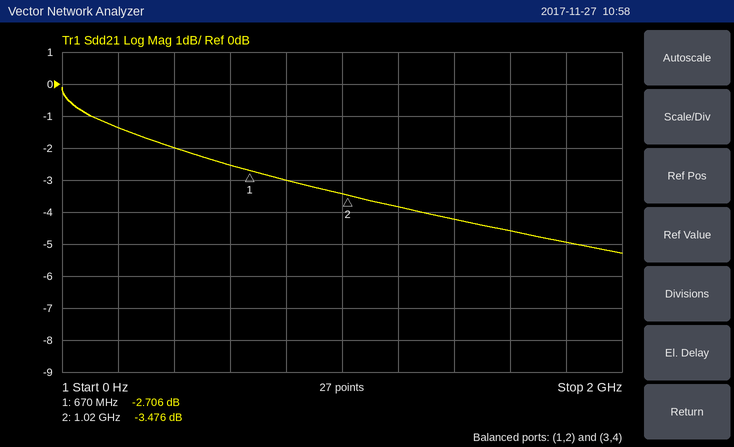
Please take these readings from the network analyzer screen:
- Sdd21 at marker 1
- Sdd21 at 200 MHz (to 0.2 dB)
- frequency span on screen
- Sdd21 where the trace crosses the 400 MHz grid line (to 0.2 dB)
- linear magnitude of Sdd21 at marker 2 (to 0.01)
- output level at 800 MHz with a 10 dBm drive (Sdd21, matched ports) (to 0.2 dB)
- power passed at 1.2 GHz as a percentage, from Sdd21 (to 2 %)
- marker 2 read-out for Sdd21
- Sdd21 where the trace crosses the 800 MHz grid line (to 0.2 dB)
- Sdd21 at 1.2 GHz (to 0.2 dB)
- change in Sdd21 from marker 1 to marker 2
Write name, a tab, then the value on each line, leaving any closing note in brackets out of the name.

Sdd21 at marker 1	-2.706 dB
Sdd21 at 200 MHz	-1.4 dB
frequency span on screen	2 GHz
Sdd21 where the trace crosses the 400 MHz grid line	-2.0 dB
linear magnitude of Sdd21 at marker 2	0.67
output level at 800 MHz with a 10 dBm drive (Sdd21, matched ports)	7.0 dBm
power passed at 1.2 GHz as a percentage, from Sdd21	42 %
marker 2 read-out for Sdd21	-3.476 dB
Sdd21 where the trace crosses the 800 MHz grid line	-3.0 dB
Sdd21 at 1.2 GHz	-3.8 dB
change in Sdd21 from marker 1 to marker 2	-0.770 dB
